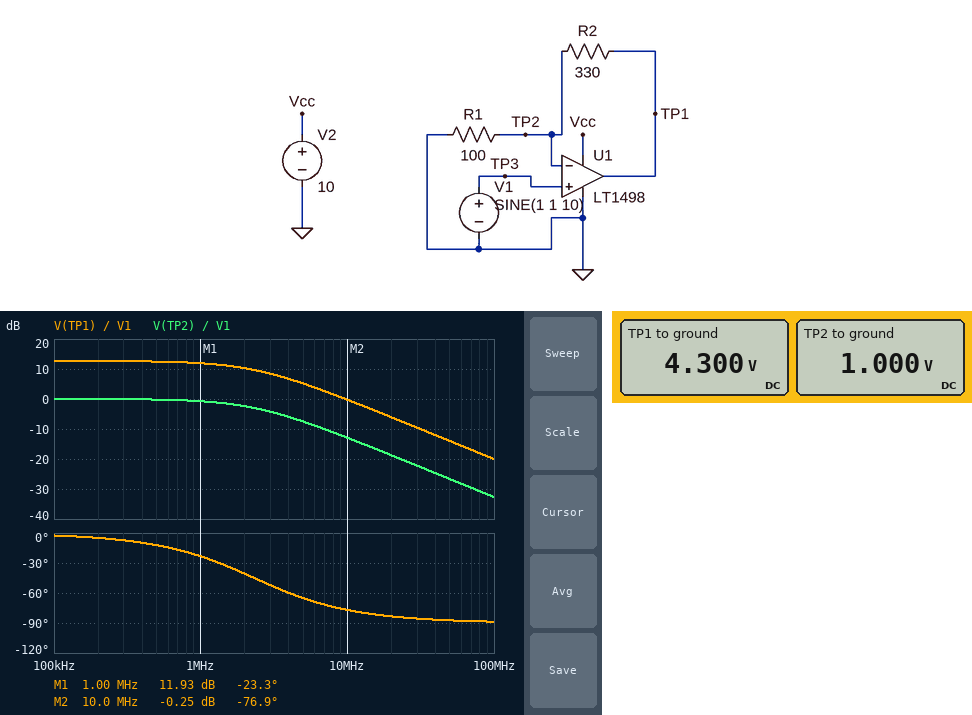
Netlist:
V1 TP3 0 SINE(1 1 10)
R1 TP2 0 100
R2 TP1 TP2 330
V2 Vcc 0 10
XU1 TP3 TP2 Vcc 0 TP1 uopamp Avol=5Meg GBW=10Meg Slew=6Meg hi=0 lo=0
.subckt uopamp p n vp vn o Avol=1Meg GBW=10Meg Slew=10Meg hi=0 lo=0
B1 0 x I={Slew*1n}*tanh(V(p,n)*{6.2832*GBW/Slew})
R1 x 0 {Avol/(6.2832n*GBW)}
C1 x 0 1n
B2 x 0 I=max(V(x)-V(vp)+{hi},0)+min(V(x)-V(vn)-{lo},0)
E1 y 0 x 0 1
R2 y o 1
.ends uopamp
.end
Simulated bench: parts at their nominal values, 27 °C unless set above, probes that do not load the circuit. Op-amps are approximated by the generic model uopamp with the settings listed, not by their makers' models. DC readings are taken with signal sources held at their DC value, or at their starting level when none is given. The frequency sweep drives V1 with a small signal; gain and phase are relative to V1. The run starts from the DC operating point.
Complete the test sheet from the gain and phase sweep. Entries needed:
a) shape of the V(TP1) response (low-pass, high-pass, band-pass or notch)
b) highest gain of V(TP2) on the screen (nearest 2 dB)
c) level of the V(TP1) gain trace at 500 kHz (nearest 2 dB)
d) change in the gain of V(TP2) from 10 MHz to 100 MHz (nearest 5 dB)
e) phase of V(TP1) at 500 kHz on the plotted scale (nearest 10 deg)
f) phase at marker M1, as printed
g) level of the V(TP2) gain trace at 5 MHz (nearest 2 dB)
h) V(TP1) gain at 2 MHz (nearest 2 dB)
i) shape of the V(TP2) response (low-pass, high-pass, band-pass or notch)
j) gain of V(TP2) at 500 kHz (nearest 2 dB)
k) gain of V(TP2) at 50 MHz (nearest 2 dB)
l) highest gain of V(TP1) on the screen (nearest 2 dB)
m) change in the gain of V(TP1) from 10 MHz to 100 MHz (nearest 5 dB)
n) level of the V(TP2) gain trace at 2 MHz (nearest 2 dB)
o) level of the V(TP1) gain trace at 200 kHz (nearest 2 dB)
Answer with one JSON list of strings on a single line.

["low-pass", "0 dB", "12 dB", "-20 dB", "-10 deg", "-23.3 deg", "-8 dB", "10 dB", "low-pass", "0 dB", "-26 dB", "12 dB", "-20 dB", "-2 dB", "12 dB"]
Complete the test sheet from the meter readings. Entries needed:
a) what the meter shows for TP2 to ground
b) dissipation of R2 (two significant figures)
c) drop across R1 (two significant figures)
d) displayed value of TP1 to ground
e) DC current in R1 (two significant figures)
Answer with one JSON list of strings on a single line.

["1.000 V", "33 mW", "1.0 V", "4.300 V", "10 mA"]
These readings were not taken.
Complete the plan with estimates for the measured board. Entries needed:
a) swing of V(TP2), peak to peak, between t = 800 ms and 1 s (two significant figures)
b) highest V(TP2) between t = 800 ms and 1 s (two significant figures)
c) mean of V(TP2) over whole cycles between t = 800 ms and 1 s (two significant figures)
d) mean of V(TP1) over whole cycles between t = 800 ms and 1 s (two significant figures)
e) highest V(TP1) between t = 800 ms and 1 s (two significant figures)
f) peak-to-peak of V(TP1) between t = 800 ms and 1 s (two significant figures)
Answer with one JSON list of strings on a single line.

["2.0 V", "2.0 V", "1.0 V", "4.3 V", "8.6 V", "8.6 V"]
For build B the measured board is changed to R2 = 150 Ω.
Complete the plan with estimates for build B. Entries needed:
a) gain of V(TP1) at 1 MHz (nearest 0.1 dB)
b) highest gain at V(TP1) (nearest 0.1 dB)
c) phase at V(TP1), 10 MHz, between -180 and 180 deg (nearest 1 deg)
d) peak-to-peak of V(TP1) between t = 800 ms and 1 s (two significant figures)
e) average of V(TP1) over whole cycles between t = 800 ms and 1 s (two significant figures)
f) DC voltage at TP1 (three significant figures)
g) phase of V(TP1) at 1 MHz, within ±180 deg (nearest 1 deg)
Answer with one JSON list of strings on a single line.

["7.7 dB", "8.0 dB", "-68 deg", "5.0 V", "2.5 V", "2.50 V", "-14 deg"]
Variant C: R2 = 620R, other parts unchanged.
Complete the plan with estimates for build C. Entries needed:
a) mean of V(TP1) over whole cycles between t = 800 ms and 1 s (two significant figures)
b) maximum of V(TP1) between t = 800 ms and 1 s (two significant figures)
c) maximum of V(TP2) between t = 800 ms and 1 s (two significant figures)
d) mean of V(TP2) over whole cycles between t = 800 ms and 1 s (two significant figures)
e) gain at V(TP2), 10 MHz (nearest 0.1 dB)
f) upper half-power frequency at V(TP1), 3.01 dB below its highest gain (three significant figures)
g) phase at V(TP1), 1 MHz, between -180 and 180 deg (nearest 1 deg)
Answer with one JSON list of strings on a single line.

["6.1 V", "10 V", "1.4 V", "850 mV", "-17.2 dB", "1.39 MHz", "-36 deg"]
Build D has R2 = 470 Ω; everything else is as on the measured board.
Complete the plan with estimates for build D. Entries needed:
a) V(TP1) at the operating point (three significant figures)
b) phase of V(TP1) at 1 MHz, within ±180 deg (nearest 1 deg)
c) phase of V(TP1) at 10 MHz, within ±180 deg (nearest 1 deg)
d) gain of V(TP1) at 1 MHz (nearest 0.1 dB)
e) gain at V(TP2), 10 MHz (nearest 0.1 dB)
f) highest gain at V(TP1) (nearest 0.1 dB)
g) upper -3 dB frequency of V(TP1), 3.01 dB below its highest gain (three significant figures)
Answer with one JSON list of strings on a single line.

["5.70 V", "-30 deg", "-80 deg", "13.9 dB", "-15.3 dB", "15.1 dB", "1.75 MHz"]
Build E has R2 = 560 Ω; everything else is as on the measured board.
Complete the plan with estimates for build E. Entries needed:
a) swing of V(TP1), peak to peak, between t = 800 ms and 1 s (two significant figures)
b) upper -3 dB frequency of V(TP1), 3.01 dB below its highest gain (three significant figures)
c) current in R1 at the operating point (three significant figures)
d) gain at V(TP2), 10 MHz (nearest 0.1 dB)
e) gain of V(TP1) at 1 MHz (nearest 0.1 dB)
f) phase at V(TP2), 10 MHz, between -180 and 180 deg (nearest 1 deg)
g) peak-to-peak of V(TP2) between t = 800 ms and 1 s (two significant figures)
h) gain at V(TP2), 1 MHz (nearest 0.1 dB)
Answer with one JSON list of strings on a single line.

["10 V", "1.51 MHz", "10.0 mA", "-16.5 dB", "14.8 dB", "-81 deg", "1.5 V", "-1.6 dB"]
